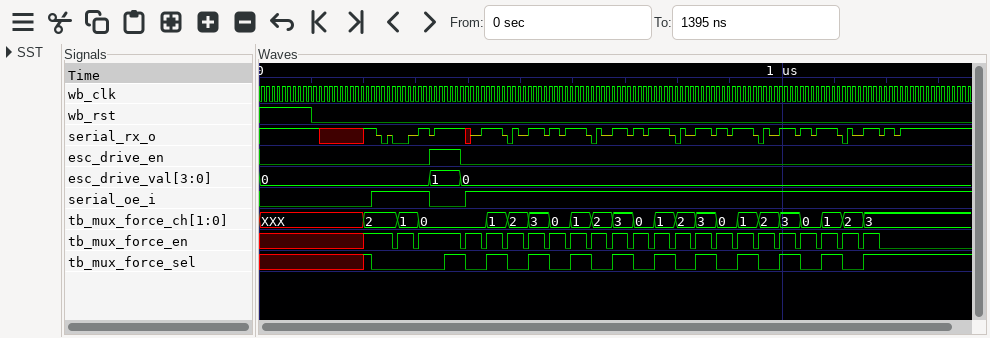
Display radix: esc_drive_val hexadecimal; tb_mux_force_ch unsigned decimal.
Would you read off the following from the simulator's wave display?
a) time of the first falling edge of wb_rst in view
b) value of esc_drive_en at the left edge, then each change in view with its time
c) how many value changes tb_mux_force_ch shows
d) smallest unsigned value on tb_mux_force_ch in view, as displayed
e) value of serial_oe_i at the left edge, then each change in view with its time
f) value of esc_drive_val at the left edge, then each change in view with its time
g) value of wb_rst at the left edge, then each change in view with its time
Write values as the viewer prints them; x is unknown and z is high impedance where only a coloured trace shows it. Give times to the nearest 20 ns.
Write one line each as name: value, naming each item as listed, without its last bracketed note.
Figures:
time of the first falling edge of wb_rst in view: 100 ns
value of esc_drive_en at the left edge, then each change in view with its time: 0, 1 at 320 ns, 0 at 380 ns
how many value changes tb_mux_force_ch shows: 22
smallest unsigned value on tb_mux_force_ch in view, as displayed: 0
value of serial_oe_i at the left edge, then each change in view with its time: 0, 1 at 220 ns, 0 at 320 ns, 1 at 400 ns
value of esc_drive_val at the left edge, then each change in view with its time: 0, 1 at 320 ns, 0 at 380 ns
value of wb_rst at the left edge, then each change in view with its time: 1, 0 at 100 ns
